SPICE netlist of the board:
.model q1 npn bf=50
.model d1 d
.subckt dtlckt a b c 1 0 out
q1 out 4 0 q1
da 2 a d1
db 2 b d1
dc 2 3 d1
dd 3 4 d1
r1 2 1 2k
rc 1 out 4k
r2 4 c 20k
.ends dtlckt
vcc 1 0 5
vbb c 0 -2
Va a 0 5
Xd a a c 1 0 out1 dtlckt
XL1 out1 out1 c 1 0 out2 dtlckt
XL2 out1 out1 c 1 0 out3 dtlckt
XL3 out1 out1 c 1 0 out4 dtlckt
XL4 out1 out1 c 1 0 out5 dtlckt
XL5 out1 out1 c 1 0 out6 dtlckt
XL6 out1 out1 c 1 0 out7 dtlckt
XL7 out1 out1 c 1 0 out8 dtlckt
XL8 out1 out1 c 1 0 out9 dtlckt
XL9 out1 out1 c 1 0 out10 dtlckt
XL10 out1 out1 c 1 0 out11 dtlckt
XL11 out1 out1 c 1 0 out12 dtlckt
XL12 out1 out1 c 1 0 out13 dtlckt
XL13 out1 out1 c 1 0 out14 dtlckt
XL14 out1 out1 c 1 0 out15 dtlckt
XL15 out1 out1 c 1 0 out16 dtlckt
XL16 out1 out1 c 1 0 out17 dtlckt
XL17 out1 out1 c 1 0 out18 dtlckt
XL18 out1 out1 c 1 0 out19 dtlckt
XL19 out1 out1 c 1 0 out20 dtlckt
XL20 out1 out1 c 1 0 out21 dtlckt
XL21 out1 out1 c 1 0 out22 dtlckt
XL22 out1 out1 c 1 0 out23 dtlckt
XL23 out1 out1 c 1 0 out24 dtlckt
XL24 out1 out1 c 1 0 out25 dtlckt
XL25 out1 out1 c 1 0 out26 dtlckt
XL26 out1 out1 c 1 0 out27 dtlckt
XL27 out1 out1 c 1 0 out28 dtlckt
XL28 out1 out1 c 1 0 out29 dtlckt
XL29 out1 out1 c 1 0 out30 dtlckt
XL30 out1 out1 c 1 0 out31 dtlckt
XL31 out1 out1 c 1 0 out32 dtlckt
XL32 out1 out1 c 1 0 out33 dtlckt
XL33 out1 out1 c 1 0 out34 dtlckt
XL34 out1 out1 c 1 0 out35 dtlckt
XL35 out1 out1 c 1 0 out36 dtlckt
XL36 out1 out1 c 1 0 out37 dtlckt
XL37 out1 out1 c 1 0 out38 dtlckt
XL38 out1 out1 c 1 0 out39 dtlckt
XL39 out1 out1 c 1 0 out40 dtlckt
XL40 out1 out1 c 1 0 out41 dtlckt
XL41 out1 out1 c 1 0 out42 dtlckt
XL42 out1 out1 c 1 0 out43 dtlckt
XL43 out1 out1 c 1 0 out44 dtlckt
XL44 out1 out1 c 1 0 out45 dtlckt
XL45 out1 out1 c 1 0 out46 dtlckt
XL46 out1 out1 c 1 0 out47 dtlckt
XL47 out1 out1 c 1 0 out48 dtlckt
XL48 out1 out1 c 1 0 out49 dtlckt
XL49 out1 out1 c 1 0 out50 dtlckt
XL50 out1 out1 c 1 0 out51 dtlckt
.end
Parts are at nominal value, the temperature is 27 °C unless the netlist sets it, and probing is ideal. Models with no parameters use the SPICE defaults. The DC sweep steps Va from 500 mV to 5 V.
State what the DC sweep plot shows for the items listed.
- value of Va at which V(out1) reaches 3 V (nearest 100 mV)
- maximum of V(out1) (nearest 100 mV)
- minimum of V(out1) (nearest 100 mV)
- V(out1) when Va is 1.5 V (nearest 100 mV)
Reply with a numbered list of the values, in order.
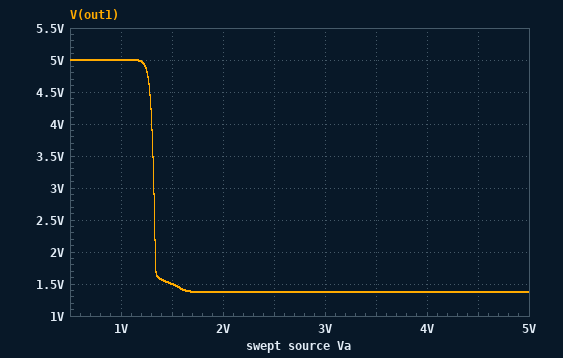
1. 1.3 V
2. 5.0 V
3. 1.4 V
4. 1.5 V
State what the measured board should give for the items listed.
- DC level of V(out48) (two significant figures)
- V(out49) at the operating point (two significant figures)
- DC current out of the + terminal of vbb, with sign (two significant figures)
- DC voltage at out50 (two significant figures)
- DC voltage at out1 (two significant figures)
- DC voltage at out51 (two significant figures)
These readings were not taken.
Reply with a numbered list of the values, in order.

1. 72 mV
2. 72 mV
3. -7.1 mA
4. 72 mV
5. 1.4 V
6. 72 mV
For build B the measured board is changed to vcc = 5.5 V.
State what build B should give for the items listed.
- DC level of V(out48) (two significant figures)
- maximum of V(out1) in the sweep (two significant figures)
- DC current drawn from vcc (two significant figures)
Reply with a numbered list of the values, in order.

1. 73 mV
2. 5.5 V
3. 160 mA
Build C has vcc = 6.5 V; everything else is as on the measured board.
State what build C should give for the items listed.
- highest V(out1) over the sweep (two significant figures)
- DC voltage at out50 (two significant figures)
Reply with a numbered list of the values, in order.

1. 6.5 V
2. 75 mV
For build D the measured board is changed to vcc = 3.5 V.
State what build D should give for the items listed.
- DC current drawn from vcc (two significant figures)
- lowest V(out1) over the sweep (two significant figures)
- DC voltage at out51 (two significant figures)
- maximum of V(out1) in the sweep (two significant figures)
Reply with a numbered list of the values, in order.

1. 81 mA
2. 1.4 V
3. 70 mV
4. 3.5 V
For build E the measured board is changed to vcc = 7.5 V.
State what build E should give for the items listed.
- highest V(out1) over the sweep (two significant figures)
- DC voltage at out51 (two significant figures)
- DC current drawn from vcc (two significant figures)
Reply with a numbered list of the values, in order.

1. 7.5 V
2. 77 mV
3. 230 mA
